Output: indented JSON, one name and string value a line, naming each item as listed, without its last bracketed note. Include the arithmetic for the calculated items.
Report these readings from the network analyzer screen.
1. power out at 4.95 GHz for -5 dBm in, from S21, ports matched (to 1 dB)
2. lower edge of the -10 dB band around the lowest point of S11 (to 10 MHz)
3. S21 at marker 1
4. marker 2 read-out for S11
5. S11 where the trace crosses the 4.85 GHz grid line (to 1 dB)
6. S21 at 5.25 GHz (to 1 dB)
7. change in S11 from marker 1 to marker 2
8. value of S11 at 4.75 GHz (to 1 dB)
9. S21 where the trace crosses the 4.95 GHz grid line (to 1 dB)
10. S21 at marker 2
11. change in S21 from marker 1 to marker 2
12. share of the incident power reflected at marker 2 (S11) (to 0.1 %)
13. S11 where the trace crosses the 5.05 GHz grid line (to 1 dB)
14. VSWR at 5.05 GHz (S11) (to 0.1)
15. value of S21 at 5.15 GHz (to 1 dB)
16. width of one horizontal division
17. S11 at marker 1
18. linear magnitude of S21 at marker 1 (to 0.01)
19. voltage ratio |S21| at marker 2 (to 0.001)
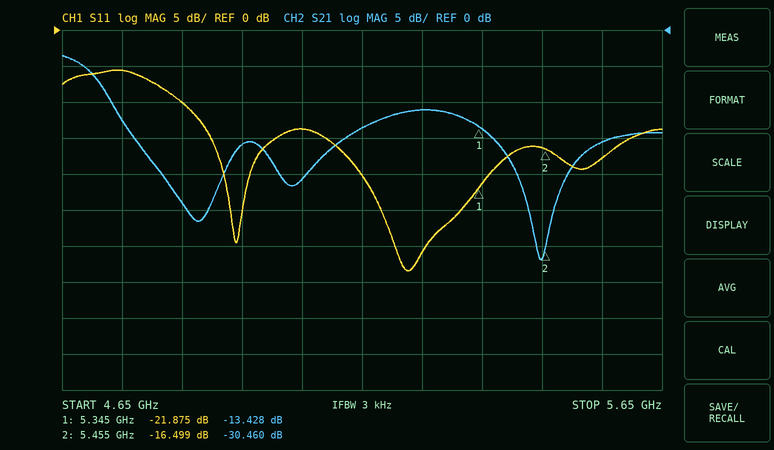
{
  "power out at 4.95 GHz for -5 dBm in, from S21, ports matched": "-5 dBm + (-16 dB) = -21 dBm",
  "lower edge of the -10 dB band around the lowest point of S11": "4.85 GHz",
  "S21 at marker 1": "-13.428 dB",
  "marker 2 read-out for S11": "-16.499 dB",
  "S11 where the trace crosses the 4.85 GHz grid line": "-10 dB",
  "S21 at 5.25 GHz": "-11 dB",
  "change in S11 from marker 1 to marker 2": "-16.499 − (-21.875) = 5.376 dB",
  "value of S11 at 4.75 GHz": "-6 dB",
  "S21 where the trace crosses the 4.95 GHz grid line": "-16 dB",
  "S21 at marker 2": "-30.460 dB",
  "change in S21 from marker 1 to marker 2": "-30.46 − (-13.428) = -17.032 dB",
  "share of the incident power reflected at marker 2 (S11)": "10^(-16.499/10) ≈ 2.2 %",
  "S11 where the trace crosses the 5.05 GHz grid line": "-14 dB",
  "VSWR at 5.05 GHz (S11)": "|Γ| = 10^(-14/20) = 0.1995; VSWR = (1 + 0.1995)/(1 − 0.1995) ≈ 1.5",
  "value of S21 at 5.15 GHz": "-14 dB",
  "width of one horizontal division": "100 MHz",
  "S11 at marker 1": "-21.875 dB",
  "linear magnitude of S21 at marker 1": "10^(-13.428/20) ≈ 0.21",
  "voltage ratio |S21| at marker 2": "10^(-30.46/20) ≈ 0.030"
}
